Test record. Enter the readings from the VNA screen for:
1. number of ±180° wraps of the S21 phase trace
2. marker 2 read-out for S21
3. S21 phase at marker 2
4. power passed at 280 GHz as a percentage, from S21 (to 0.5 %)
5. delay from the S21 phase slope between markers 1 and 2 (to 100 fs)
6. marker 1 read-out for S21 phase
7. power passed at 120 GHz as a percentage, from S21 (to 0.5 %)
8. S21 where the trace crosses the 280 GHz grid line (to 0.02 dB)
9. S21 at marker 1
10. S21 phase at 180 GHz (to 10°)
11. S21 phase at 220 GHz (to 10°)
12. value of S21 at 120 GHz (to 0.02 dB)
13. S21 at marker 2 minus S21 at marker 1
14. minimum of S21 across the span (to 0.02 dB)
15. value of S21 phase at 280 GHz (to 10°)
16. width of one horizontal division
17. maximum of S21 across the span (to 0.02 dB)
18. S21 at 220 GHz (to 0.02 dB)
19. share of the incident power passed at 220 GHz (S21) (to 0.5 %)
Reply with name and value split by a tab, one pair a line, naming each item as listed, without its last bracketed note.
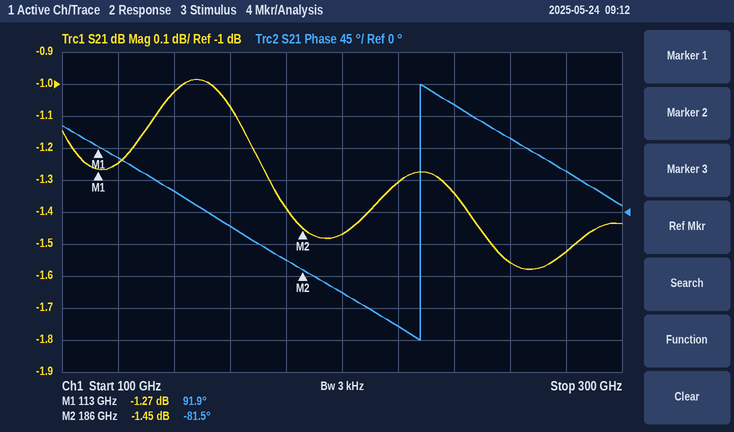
number of ±180° wraps of the S21 phase trace	1
marker 2 read-out for S21	-1.45 dB
S21 phase at marker 2	-81.5°
power passed at 280 GHz as a percentage, from S21	70.5 %
delay from the S21 phase slope between markers 1 and 2	6.6 ps
marker 1 read-out for S21 phase	91.9°
power passed at 120 GHz as a percentage, from S21	75.0 %
S21 where the trace crosses the 280 GHz grid line	-1.52 dB
S21 at marker 1	-1.27 dB
S21 phase at 180 GHz	-70°
S21 phase at 220 GHz	-160°
value of S21 at 120 GHz	-1.24 dB
S21 at marker 2 minus S21 at marker 1	-0.18 dB
minimum of S21 across the span	-1.58 dB
value of S21 phase at 280 GHz	60°
width of one horizontal division	20 GHz
maximum of S21 across the span	-0.98 dB
S21 at 220 GHz	-1.30 dB
share of the incident power passed at 220 GHz (S21)	74.0 %
